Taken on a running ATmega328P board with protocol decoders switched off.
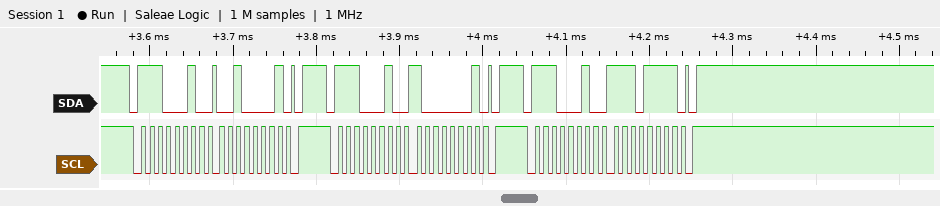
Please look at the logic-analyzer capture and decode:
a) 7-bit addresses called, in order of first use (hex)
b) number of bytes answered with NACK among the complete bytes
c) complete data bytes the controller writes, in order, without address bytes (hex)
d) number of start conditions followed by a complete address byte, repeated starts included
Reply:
0x71
0
21 81 EF
3
